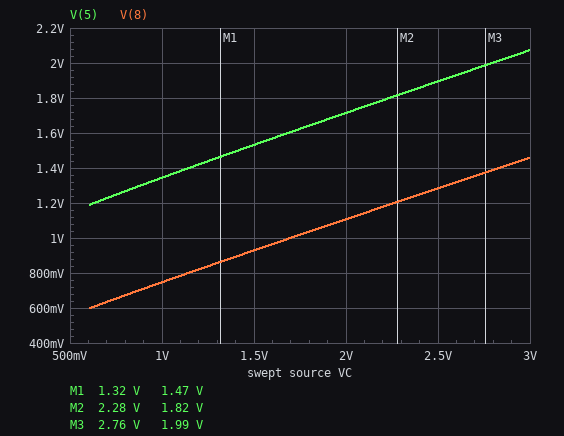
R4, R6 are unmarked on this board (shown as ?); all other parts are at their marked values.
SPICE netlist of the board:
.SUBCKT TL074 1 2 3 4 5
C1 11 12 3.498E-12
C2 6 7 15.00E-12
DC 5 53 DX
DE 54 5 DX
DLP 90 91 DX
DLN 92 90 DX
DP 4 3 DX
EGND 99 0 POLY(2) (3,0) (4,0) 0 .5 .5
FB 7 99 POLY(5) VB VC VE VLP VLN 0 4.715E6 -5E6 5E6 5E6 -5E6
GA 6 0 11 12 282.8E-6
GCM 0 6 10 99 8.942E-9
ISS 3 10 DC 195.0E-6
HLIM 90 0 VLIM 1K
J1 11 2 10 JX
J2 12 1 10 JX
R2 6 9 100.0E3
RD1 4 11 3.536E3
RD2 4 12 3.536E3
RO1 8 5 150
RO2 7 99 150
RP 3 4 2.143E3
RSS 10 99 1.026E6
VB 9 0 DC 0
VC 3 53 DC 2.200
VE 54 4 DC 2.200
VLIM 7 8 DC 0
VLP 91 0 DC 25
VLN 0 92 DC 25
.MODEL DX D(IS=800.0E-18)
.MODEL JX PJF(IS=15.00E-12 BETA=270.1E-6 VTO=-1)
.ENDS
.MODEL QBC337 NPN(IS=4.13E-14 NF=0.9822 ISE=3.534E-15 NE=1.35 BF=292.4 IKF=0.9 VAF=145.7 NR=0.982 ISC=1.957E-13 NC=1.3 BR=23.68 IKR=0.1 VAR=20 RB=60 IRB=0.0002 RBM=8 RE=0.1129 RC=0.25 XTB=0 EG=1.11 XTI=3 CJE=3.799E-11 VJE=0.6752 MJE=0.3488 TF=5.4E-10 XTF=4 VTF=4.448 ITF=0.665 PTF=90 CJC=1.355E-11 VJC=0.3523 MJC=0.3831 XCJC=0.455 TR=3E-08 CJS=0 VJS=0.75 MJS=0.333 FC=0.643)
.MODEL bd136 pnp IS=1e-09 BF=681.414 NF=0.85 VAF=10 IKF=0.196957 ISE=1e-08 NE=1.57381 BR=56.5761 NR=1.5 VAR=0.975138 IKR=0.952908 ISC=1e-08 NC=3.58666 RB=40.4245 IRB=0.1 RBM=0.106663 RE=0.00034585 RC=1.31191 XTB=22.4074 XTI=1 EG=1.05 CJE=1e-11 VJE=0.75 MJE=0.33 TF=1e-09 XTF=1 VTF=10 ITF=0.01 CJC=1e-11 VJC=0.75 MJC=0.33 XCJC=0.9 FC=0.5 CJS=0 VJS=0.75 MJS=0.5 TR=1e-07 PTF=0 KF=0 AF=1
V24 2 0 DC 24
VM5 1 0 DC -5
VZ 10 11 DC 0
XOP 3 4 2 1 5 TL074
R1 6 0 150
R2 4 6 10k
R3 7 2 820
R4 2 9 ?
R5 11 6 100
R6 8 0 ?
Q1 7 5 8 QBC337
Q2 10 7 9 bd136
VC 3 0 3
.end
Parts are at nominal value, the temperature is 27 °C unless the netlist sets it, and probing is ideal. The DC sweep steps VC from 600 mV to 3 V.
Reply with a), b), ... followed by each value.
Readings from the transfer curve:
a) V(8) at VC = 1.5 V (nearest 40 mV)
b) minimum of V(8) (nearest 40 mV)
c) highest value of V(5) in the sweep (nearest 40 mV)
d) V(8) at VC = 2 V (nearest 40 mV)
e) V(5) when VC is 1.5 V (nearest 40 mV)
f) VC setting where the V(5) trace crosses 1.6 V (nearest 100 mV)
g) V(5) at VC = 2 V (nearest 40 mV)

a) 920 mV
b) 600 mV
c) 2.08 V
d) 1.12 V
e) 1.52 V
f) 1.7 V
g) 1.72 V
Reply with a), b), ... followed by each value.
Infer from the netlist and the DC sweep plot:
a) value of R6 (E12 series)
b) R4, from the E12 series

a) 1 kΩ
b) 39 Ω
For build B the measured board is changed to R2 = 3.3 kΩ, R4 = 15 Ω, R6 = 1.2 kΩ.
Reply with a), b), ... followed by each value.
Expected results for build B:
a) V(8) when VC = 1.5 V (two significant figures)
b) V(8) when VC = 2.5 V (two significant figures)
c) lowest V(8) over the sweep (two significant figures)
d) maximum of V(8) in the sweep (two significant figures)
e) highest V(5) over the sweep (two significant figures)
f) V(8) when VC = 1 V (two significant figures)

a) 760 mV
b) 950 mV
c) 570 mV
d) 1.0 V
e) 1.6 V
f) 660 mV
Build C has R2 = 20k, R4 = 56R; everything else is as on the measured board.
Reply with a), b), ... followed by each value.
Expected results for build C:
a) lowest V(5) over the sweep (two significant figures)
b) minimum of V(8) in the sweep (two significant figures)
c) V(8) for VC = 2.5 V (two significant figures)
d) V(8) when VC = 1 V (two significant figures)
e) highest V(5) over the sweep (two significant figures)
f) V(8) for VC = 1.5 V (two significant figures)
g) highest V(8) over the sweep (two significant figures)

a) 1.3 V
b) 680 mV
c) 1.6 V
d) 890 mV
e) 2.5 V
f) 1.1 V
g) 1.9 V
